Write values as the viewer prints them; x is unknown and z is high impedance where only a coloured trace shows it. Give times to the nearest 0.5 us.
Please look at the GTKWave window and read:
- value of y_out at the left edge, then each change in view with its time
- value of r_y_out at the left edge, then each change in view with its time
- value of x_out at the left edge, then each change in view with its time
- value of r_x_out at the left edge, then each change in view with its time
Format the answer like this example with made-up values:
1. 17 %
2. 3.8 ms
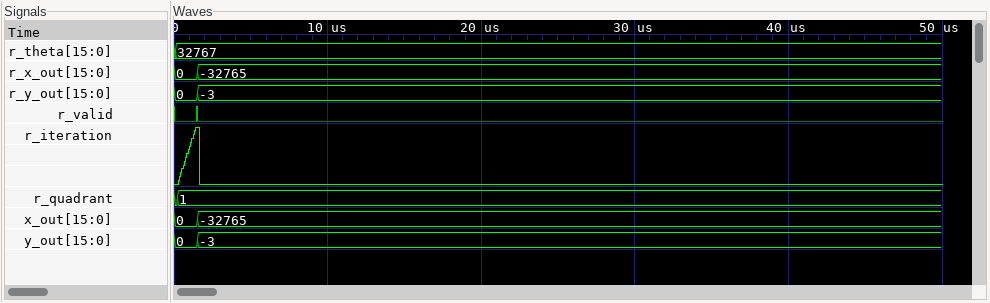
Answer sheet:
1. 0, -3 at 1.5 us
2. 0, -3 at 1.5 us
3. 0, -32765 at 1.5 us
4. 0, -32765 at 1.5 us
